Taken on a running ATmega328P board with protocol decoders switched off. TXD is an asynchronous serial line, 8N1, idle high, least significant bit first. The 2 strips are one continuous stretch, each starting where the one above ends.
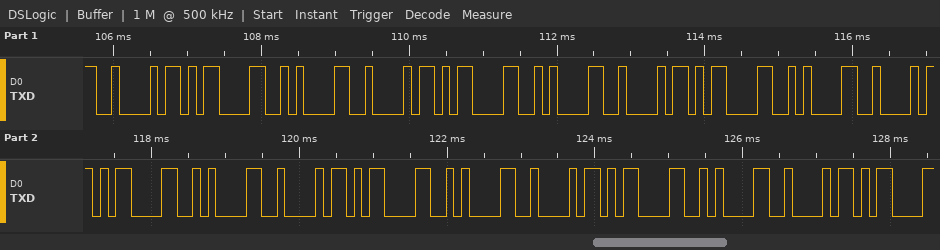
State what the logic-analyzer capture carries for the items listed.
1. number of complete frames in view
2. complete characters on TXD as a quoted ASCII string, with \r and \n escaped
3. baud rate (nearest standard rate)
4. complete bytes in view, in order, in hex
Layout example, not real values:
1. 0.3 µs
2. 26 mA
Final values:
1. 20
2. "B\r\nB\r\nB\r\nB\r\nB\r\nB\r\nB\r"
3. 9600 baud
4. 42 0D 0A 42 0D 0A 42 0D 0A 42 0D 0A 42 0D 0A 42 0D 0A 42 0D
